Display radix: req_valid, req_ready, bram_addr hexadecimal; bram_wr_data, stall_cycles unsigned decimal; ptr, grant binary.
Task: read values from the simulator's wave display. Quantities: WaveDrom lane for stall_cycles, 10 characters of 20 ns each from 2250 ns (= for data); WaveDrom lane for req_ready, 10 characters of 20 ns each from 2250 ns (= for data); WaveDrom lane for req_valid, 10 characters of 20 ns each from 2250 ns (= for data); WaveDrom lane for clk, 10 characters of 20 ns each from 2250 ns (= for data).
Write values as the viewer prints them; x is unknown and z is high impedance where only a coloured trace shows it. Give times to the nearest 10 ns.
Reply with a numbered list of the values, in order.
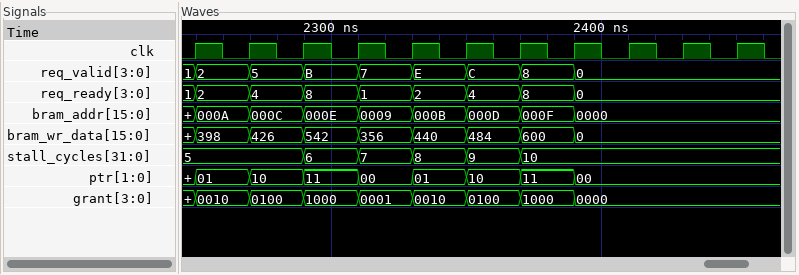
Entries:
1. {name: 'stall_cycles', wave: '=.=====...', data: '5 6 7 8 9 10'}
2. {name: 'req_ready', wave: '========..', data: '2 4 8 1 2 4 8 0'}
3. {name: 'req_valid', wave: '========..', data: '2 5 B 7 E C 8 0'}
4. {name: 'clk', wave: 'p.........'}
